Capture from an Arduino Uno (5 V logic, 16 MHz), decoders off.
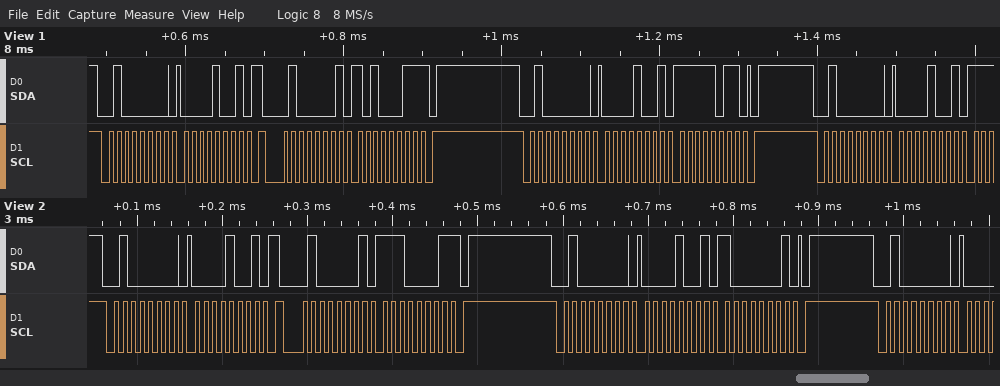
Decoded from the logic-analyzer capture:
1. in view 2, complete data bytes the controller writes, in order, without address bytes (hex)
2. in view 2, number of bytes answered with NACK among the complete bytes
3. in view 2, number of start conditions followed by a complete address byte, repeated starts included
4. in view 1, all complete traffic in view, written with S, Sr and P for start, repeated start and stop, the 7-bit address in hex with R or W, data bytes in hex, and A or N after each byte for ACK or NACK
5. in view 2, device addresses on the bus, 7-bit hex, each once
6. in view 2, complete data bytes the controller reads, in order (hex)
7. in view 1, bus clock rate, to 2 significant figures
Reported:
09 09 81
1
4
S 20W A 09 A Sr 20R A A3 N P S 20W A 09 A FB A P S 20W A 09 A
0x20
E1
100 kHz
